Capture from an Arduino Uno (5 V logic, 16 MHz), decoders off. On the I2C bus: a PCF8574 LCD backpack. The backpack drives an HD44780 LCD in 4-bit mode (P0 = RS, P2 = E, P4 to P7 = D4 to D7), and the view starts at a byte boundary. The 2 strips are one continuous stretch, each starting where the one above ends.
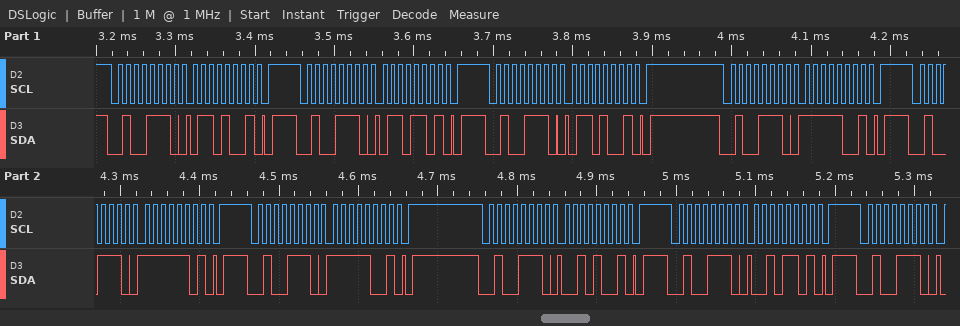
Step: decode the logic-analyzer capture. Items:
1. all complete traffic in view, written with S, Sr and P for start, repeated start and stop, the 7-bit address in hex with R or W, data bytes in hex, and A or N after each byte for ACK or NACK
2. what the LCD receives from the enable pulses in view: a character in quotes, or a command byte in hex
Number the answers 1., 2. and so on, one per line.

1. S 27W A 69 A P S 27W A 6D A P S 27W A 69 A P S 27W A F9 A P S 27W A FD A P S 27W A F9 A P S 27W A 29 A P S 27W A 2D A P S 27W A
2. 'o'
